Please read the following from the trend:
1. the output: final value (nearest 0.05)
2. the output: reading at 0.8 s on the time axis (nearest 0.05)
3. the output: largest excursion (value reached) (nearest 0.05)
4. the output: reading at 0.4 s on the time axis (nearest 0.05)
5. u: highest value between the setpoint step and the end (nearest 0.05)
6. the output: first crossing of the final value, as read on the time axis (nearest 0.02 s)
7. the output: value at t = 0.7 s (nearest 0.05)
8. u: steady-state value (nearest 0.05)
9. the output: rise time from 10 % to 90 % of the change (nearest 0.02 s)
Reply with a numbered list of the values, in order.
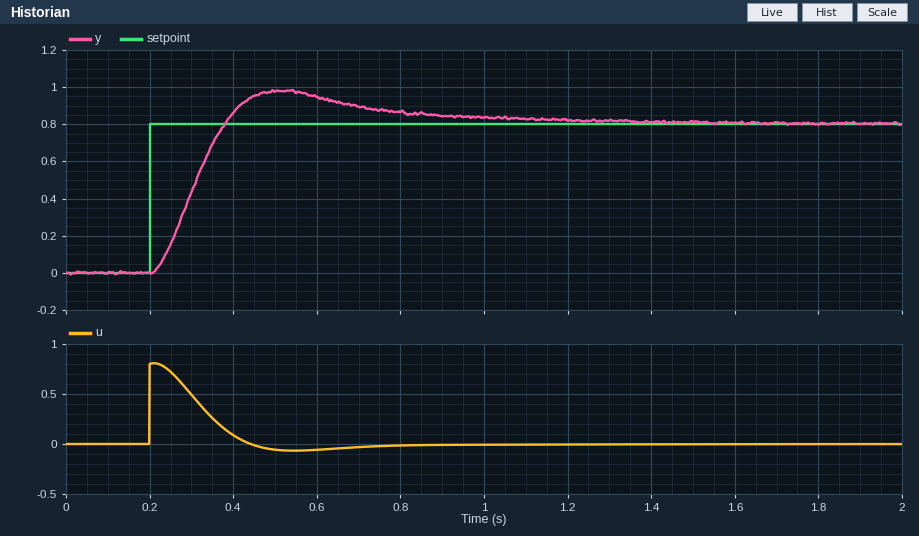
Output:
1. 0.80
2. 0.85
3. 1.00
4. 0.85
5. 0.80
6. 0.38 s
7. 0.90
8. 0.00
9. 0.12 s
